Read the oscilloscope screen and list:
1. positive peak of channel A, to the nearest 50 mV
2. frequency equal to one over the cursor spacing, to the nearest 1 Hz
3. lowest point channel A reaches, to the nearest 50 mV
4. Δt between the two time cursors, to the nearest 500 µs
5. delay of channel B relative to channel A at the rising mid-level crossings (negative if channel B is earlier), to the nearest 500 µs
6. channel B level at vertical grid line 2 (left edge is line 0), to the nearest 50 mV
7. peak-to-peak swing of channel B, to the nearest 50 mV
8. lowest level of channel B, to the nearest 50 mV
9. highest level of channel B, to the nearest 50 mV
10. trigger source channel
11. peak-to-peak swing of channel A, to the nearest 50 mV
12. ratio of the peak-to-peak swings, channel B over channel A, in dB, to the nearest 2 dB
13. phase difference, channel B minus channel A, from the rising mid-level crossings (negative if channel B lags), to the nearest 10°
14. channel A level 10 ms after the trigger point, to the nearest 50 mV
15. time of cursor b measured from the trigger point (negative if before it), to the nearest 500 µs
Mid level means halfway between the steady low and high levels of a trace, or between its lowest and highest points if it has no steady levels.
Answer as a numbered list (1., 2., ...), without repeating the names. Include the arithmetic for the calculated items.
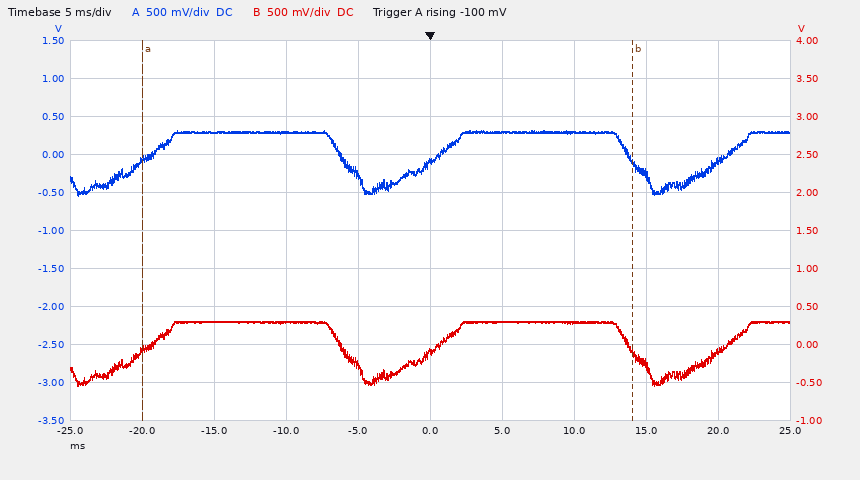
1. 300 mV
2. 1 / 34.0 ms ≈ 29 Hz
3. -550 mV
4. 34.0 ms
5. 0.0 ms
6. 300 mV
7. 300 mV − (-550 mV) = 850 mV
8. -550 mV
9. 300 mV
10. channel A
11. 300 mV − (-550 mV) = 850 mV
12. 20 log10(850 mV / 850 mV) ≈ 0 dB
13. 0°
14. 300 mV
15. +14.0 ms
